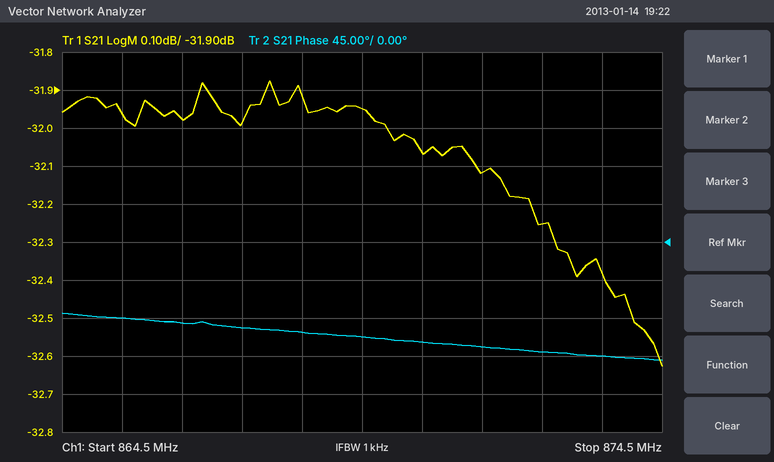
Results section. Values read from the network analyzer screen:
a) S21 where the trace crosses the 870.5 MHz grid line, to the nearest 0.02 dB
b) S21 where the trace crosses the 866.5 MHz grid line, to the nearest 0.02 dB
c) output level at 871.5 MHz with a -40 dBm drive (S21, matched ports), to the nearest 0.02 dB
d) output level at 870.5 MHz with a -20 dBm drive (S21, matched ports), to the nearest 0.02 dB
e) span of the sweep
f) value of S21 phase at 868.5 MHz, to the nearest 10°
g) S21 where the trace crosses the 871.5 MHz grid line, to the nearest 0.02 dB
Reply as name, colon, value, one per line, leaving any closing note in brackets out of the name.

S21 where the trace crosses the 870.5 MHz grid line, to the nearest 0.02 dB: -32.06 dB
S21 where the trace crosses the 866.5 MHz grid line, to the nearest 0.02 dB: -31.98 dB
output level at 871.5 MHz with a -40 dBm drive (S21, matched ports), to the nearest 0.02 dB: -72.12 dBm
output level at 870.5 MHz with a -20 dBm drive (S21, matched ports), to the nearest 0.02 dB: -52.06 dBm
span of the sweep: 10 MHz
value of S21 phase at 868.5 MHz, to the nearest 10°: -110°
S21 where the trace crosses the 871.5 MHz grid line, to the nearest 0.02 dB: -32.12 dB
